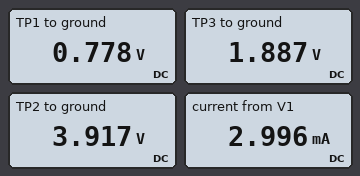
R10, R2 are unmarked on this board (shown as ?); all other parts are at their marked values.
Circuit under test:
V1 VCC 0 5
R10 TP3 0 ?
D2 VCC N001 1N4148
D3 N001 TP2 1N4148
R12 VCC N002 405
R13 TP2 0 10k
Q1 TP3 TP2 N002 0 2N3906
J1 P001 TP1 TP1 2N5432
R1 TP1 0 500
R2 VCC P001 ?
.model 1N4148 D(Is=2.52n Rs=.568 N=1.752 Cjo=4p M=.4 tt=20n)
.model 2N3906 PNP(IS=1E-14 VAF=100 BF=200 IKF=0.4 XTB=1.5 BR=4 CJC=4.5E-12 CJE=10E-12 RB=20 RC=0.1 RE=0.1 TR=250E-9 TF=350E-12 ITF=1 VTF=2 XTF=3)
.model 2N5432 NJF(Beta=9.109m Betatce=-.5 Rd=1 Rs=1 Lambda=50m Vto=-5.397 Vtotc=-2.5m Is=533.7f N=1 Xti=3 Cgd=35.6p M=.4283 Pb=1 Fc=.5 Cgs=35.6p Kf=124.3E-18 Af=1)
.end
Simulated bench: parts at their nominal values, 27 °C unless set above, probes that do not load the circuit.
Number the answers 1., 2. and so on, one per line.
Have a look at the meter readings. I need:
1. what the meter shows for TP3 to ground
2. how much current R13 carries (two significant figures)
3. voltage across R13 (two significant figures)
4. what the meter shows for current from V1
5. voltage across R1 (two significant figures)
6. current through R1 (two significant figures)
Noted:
1. 1.887 V
2. 390 µA
3. 3.9 V
4. 2.996 mA
5. 780 mV
6. 1.6 mA
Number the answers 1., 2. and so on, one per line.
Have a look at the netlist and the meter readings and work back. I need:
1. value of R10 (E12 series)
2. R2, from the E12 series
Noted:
1. 1.8 kΩ
2. 2.7 kΩ
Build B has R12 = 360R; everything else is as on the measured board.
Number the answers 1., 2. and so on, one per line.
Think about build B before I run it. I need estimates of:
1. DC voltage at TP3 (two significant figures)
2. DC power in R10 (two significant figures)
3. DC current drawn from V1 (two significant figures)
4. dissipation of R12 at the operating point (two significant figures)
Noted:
1. 2.1 V
2. 2.5 mW
3. 3.1 mA
4. 500 µW
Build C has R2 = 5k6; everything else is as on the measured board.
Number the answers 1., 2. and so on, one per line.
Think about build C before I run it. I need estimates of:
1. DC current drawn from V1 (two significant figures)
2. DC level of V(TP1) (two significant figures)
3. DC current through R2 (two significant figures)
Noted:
1. 2.3 mA
2. 410 mV
3. 820 µA
